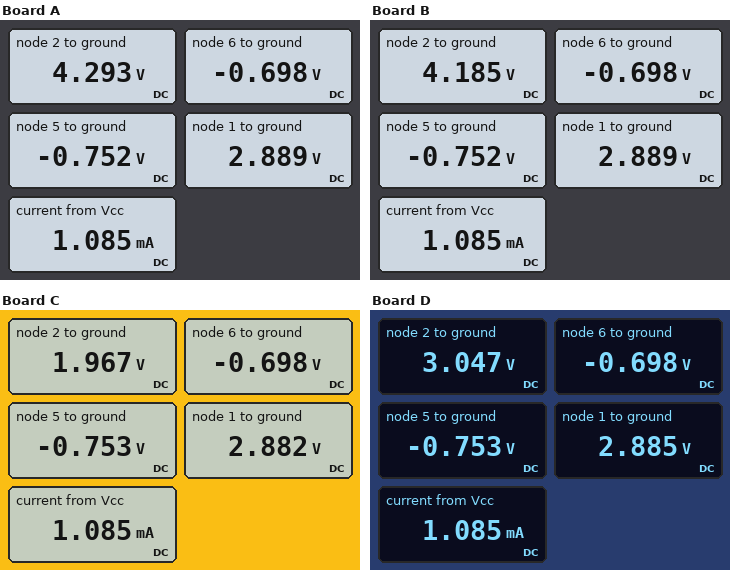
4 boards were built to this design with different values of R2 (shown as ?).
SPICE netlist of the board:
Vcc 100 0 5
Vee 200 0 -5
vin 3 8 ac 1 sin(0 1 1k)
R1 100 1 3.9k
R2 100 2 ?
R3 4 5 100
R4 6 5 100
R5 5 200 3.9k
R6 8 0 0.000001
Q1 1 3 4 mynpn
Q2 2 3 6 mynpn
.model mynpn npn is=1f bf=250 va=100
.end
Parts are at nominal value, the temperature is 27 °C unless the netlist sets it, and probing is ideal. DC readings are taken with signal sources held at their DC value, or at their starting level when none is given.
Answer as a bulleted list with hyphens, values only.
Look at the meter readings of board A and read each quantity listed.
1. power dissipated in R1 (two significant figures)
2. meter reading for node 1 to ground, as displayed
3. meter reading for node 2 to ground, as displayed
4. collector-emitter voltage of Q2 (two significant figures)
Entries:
- 1.1 mW
- 2.889 V
- 4.293 V
- 5.0 V
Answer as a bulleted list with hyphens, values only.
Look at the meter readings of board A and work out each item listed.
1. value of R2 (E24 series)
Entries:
- 1.3 kΩ
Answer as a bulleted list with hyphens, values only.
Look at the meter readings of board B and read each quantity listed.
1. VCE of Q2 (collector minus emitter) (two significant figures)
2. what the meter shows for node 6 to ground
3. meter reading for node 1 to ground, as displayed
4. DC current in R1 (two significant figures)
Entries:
- 4.9 V
- -0.698 V
- 2.889 V
- 540 µA
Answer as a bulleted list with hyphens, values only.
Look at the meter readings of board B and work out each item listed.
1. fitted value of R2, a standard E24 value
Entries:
- 1.5 kΩ
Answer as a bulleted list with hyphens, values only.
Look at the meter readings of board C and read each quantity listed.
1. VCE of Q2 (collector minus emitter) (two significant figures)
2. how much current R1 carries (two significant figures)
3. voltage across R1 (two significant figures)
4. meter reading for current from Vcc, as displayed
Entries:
- 2.7 V
- 540 µA
- 2.1 V
- 1.085 mA
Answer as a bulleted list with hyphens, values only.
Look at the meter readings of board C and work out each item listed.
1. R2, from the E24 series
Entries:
- 5.6 kΩ
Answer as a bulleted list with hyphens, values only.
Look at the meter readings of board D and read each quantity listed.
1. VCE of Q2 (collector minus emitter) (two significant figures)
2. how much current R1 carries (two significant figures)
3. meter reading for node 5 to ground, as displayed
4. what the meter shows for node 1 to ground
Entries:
- 3.7 V
- 540 µA
- -0.753 V
- 2.885 V
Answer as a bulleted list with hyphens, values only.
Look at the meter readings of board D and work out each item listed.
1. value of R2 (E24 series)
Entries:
- 3.6 kΩ
